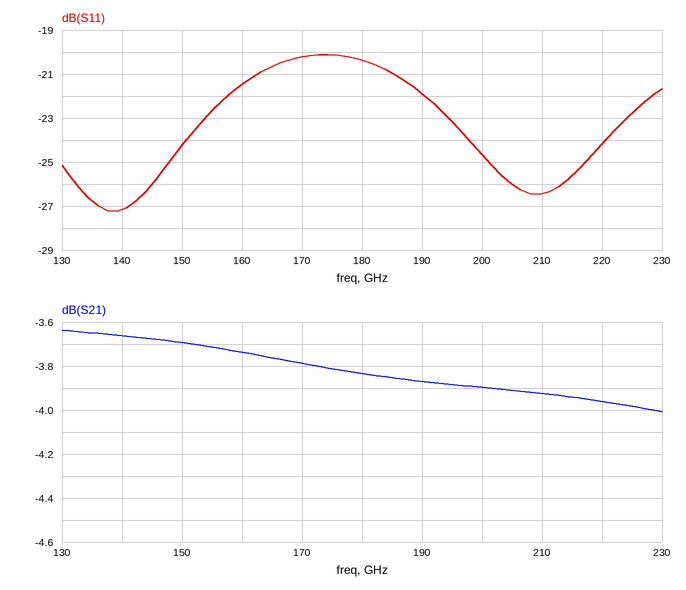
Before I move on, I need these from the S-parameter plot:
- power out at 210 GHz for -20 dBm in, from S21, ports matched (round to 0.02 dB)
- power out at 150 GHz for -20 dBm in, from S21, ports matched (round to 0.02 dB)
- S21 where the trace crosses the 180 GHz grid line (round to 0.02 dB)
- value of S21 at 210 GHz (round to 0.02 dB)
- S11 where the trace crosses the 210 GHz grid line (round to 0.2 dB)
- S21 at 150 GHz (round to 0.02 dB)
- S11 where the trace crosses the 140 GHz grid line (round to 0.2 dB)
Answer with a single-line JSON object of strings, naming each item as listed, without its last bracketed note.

{"power out at 210 GHz for -20 dBm in, from S21, ports matched": "-23.92 dBm", "power out at 150 GHz for -20 dBm in, from S21, ports matched": "-23.70 dBm", "S21 where the trace crosses the 180 GHz grid line": "-3.84 dB", "value of S21 at 210 GHz": "-3.92 dB", "S11 where the trace crosses the 210 GHz grid line": "-26.4 dB", "S21 at 150 GHz": "-3.70 dB", "S11 where the trace crosses the 140 GHz grid line": "-27.2 dB"}
